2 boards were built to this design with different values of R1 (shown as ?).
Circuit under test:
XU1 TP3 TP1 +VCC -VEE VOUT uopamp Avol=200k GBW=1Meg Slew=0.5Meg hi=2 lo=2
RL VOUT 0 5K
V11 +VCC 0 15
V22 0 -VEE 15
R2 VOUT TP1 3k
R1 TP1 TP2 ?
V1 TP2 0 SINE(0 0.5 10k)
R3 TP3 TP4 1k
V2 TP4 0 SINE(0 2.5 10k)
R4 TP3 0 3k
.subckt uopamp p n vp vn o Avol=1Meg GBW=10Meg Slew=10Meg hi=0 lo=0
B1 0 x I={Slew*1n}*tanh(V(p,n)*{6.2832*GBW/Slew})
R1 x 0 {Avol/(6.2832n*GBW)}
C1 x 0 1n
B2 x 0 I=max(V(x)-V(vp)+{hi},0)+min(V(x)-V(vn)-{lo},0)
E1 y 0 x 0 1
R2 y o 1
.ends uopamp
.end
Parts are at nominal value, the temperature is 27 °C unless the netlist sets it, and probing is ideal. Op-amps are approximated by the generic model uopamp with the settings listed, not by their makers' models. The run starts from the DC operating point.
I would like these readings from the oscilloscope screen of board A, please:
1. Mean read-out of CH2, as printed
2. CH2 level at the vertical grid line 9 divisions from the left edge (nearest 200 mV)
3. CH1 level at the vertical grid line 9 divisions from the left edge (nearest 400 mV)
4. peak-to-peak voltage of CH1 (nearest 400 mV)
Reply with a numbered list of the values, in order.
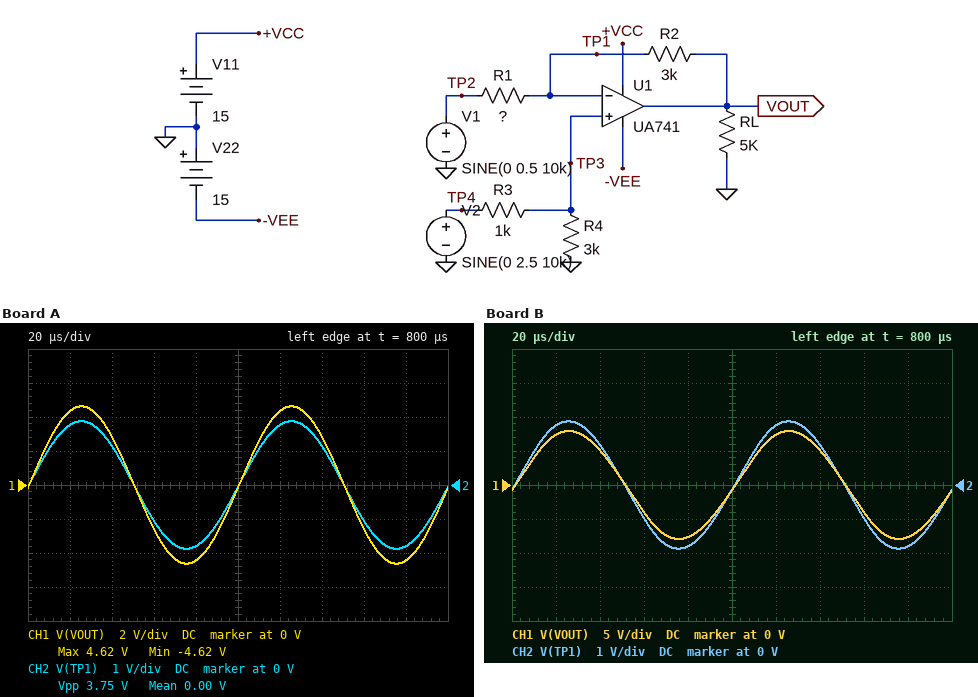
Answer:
1. 0.00 V
2. -1.8 V
3. -4.4 V
4. 9.2 V
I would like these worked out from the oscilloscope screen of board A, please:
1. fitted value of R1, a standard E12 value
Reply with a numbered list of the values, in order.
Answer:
1. 1.5 kΩ
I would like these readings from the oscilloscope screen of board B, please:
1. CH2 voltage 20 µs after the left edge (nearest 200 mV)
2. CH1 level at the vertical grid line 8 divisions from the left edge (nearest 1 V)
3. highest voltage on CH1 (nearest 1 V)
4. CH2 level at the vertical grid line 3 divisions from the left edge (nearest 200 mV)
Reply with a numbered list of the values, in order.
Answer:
1. 1.8 V
2. -4 V
3. 8 V
4. -1.0 V
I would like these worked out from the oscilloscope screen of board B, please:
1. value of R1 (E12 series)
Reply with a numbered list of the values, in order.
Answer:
1. 680 Ω
